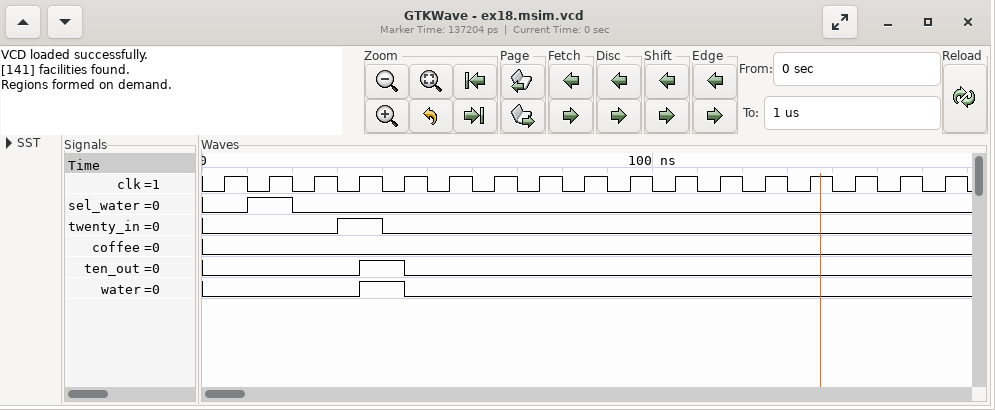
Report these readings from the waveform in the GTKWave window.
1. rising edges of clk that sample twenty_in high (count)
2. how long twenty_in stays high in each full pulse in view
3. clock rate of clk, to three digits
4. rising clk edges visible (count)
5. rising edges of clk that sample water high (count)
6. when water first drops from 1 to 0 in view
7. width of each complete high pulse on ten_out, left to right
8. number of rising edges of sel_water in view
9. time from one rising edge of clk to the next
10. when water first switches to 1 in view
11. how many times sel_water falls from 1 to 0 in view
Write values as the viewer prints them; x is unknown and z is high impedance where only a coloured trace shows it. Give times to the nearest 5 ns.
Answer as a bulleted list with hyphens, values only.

- 1
- 10 ns
- 100 MHz
- 17
- 1
- 45 ns
- 10 ns
- 1
- 10 ns
- 35 ns
- 1
